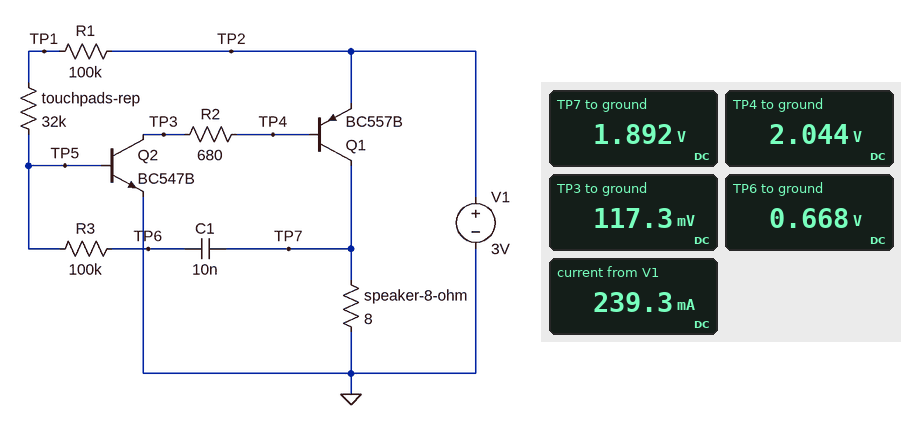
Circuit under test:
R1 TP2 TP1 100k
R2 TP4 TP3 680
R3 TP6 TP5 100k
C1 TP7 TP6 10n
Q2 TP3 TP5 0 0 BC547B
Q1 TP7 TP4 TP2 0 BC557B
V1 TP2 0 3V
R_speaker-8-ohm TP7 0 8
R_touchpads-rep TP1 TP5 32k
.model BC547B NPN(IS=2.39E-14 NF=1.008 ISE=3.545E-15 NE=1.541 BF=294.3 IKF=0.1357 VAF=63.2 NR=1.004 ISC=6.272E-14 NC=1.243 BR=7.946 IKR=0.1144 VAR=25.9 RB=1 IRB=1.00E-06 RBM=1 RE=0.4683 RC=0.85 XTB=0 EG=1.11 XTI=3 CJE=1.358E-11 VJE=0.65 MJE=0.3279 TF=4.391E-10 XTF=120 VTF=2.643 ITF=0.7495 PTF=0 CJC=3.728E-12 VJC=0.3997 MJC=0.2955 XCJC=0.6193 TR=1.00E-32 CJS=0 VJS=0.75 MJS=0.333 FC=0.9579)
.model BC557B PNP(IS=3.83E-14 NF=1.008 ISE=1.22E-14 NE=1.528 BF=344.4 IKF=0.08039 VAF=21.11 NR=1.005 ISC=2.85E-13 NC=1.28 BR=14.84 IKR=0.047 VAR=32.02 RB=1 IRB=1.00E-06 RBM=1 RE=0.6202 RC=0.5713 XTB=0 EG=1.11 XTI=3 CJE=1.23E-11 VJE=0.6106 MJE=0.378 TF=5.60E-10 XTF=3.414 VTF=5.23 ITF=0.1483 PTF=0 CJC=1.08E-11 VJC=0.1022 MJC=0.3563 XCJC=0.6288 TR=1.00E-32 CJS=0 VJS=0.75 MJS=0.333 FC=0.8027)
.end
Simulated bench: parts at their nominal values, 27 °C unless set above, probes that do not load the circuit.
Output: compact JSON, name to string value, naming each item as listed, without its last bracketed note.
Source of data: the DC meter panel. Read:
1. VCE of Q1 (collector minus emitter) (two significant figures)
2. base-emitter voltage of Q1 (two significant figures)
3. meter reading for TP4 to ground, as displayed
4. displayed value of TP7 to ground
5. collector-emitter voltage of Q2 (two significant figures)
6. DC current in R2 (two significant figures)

{"VCE of Q1 (collector minus emitter)": "-1.1 V", "base-emitter voltage of Q1": "-960 mV", "meter reading for TP4 to ground, as displayed": "2.044 V", "displayed value of TP7 to ground": "1.892 V", "collector-emitter voltage of Q2": "120 mV", "DC current in R2": "2.8 mA"}
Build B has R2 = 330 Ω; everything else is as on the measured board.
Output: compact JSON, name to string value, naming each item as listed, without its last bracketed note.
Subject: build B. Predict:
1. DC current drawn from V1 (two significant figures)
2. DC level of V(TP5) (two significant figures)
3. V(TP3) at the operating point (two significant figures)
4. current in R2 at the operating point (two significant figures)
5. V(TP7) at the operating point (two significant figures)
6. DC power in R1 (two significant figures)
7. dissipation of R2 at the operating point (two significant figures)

{"DC current drawn from V1": "310 mA", "DC level of V(TP5)": "680 mV", "V(TP3) at the operating point": "400 mV", "current in R2 at the operating point": "4.8 mA", "V(TP7) at the operating point": "2.4 V", "DC power in R1": "31 µW", "dissipation of R2 at the operating point": "7.6 mW"}
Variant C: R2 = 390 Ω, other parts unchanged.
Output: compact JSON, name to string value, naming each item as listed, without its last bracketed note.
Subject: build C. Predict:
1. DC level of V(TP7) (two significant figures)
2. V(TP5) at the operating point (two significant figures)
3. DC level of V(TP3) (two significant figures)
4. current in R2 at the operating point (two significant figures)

{"DC level of V(TP7)": "2.4 V", "V(TP5) at the operating point": "680 mV", "DC level of V(TP3)": "200 mV", "current in R2 at the operating point": "4.6 mA"}
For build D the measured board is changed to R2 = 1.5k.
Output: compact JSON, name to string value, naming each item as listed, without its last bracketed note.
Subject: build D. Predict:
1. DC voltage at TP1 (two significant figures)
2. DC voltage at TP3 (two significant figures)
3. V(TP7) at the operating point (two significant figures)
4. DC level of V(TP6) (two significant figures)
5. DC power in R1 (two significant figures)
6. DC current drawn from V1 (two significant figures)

{"DC voltage at TP1": "1.2 V", "DC voltage at TP3": "82 mV", "V(TP7) at the operating point": "1.3 V", "DC level of V(TP6)": "650 mV", "DC power in R1": "32 µW", "DC current drawn from V1": "160 mA"}
